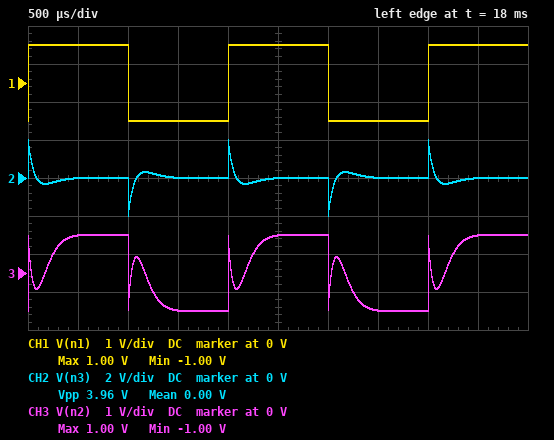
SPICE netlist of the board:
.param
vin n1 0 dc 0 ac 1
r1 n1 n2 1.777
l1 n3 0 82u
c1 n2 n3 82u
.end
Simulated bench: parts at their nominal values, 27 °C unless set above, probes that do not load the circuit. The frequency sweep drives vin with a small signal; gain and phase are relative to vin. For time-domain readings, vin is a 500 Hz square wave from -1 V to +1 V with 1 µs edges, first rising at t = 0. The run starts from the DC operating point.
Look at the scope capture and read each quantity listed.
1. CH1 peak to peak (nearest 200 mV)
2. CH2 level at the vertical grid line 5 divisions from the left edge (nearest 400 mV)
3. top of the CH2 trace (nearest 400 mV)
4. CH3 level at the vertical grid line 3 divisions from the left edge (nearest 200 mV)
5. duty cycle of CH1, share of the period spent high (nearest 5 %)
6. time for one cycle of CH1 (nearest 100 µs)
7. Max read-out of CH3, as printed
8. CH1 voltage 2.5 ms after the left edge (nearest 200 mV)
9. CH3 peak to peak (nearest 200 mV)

2.0 V
0 V
2.0 V
-1.0 V
50 %
2.0 ms
1.00 V
1.0 V
2.0 V
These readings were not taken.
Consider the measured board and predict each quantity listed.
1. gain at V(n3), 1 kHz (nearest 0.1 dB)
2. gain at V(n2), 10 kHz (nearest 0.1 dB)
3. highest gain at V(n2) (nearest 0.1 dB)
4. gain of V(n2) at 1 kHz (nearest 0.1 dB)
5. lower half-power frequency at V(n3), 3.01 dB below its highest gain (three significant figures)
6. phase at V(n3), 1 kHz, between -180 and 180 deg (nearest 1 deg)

-12.9 dB
-0.5 dB
0 dB
-4.1 dB
2.56 kHz
129 deg
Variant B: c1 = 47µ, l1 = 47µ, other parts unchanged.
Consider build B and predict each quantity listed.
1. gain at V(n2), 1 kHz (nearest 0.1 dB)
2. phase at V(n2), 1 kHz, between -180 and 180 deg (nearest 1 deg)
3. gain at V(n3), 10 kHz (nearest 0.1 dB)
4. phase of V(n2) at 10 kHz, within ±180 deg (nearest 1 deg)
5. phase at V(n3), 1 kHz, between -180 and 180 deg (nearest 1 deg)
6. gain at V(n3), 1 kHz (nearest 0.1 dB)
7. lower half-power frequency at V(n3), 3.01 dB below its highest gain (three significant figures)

-1.2 dB
-30 deg
-0.6 dB
34 deg
150 deg
-21.6 dB
4.46 kHz
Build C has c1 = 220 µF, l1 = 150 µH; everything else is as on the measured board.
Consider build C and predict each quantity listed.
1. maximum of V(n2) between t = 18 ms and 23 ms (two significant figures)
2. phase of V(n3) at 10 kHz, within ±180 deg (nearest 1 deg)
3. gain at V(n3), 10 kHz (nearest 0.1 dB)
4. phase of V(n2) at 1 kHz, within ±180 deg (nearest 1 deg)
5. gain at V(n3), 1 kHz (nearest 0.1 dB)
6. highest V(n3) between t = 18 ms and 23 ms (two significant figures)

1.1 V
11 deg
-0.1 dB
83 deg
-5.6 dB
2.0 V
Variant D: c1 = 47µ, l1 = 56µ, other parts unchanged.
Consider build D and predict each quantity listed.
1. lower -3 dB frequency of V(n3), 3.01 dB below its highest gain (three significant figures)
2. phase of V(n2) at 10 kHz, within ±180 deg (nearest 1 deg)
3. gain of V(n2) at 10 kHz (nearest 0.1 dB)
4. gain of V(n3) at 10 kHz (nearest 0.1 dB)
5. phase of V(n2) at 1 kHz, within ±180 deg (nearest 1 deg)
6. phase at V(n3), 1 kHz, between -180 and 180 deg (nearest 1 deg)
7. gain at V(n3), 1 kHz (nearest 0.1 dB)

3.64 kHz
29 deg
-1.2 dB
-0.3 dB
-30 deg
150 deg
-20.0 dB
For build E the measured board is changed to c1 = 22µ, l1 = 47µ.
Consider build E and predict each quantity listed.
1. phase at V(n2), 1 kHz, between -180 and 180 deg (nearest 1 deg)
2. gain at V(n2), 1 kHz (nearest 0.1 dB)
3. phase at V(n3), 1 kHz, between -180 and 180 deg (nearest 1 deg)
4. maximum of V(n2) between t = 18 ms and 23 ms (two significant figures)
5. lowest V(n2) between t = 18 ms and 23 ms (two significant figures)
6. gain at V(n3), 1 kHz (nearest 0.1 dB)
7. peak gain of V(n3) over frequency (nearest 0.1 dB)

-14 deg
-0.3 dB
166 deg
1.1 V
-1.1 V
-27.7 dB
0.3 dB
